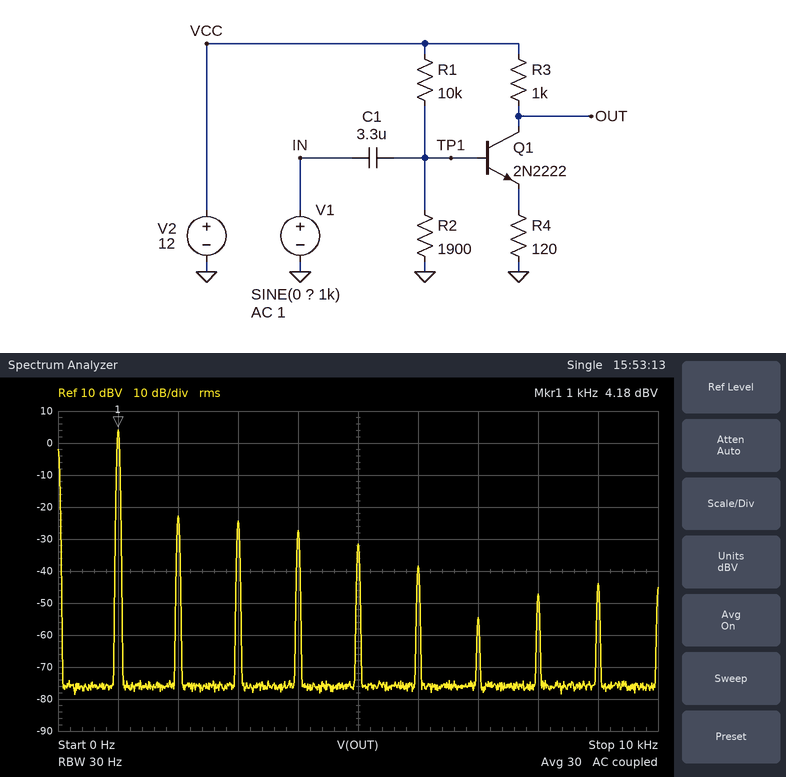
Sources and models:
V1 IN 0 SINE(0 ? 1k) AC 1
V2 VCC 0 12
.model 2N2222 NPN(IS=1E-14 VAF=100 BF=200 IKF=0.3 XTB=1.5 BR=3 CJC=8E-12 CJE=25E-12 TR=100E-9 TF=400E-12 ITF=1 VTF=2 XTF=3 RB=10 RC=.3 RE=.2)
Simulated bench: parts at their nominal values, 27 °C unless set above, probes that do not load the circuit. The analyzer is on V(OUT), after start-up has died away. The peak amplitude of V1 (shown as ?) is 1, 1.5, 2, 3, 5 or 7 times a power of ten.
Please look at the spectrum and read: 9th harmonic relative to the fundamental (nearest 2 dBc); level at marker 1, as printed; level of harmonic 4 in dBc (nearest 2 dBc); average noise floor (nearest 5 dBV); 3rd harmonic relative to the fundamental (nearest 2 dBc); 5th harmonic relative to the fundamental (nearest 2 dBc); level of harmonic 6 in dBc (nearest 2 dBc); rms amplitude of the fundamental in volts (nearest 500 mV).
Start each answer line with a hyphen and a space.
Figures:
- -48 dBc
- 4.18 dBV
- -32 dBc
- -75 dBV
- -28 dBc
- -36 dBc
- -42 dBc
- 1.5 V
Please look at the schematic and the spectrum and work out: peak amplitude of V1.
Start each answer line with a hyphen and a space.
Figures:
- 300 mV
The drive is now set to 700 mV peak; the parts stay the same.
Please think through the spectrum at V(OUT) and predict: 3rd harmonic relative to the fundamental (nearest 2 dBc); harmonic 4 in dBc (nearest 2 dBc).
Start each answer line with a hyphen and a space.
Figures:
- -24 dBc
- -30 dBc
